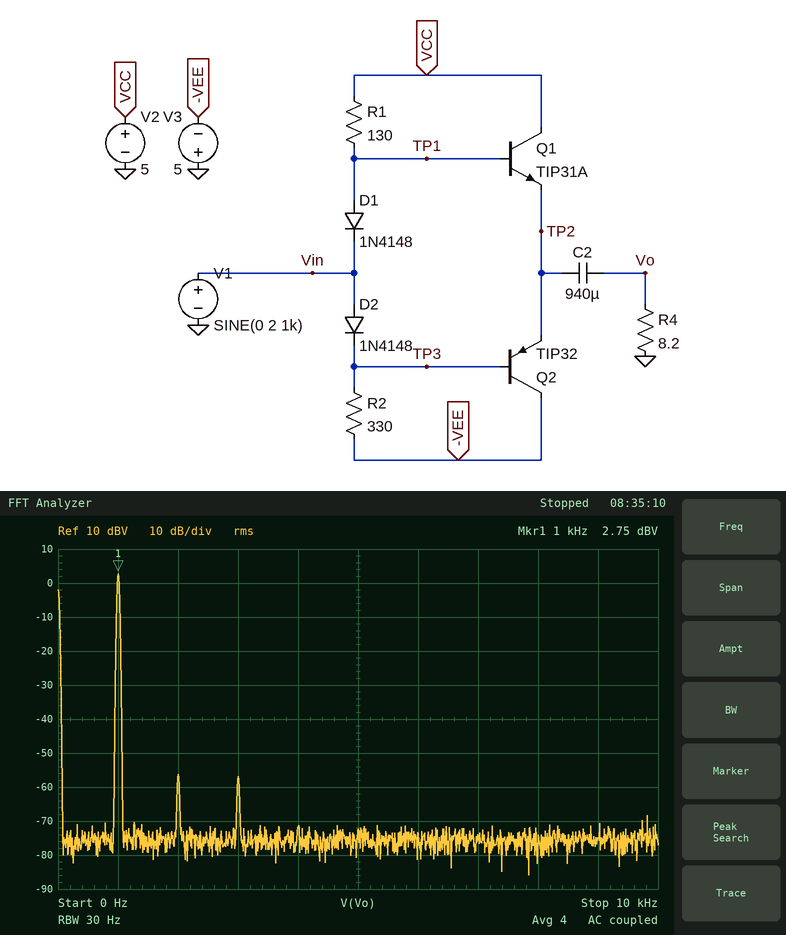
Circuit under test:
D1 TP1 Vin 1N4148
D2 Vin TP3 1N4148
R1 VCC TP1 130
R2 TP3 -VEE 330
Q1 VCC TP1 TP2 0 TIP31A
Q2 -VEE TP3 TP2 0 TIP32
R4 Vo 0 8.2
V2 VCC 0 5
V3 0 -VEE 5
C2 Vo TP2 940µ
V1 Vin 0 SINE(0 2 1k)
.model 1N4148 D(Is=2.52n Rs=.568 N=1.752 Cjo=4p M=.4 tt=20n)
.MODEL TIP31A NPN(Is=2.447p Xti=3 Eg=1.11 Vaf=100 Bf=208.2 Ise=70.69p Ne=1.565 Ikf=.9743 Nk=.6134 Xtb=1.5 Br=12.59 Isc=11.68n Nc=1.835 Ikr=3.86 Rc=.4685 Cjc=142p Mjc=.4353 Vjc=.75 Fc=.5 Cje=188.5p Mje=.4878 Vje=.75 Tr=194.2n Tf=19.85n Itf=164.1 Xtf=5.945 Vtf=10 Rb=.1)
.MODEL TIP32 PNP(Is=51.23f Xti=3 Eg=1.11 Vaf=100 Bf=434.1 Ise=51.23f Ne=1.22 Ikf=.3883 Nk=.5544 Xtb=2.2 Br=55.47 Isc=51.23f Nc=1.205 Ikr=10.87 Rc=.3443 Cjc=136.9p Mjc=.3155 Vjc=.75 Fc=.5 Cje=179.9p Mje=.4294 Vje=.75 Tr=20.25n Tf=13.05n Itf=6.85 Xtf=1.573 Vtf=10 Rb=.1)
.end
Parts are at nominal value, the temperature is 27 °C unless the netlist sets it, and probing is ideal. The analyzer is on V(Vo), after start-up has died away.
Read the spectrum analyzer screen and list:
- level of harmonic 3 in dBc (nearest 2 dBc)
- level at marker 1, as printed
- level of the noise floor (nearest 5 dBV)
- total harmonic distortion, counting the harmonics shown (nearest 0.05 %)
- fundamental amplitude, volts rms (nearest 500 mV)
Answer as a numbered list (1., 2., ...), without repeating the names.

1. -60 dBc
2. 2.75 dBV
3. -75 dBV
4. 0.15 %
5. 1.5 V
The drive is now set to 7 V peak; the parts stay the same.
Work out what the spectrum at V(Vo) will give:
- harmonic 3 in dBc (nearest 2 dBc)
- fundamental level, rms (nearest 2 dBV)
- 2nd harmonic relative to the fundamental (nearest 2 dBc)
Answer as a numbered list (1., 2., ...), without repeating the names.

1. -12 dBc
2. 8 dBV
3. -24 dBc
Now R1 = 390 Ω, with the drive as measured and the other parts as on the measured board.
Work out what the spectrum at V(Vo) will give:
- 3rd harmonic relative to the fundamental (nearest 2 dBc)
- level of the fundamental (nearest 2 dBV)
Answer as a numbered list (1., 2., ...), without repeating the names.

1. -54 dBc
2. 2 dBV
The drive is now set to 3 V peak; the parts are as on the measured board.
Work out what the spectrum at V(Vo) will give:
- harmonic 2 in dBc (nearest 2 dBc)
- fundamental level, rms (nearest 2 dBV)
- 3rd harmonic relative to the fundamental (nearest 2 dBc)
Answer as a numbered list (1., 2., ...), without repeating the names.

1. -42 dBc
2. 6 dBV
3. -42 dBc
